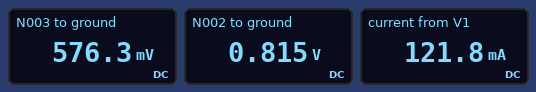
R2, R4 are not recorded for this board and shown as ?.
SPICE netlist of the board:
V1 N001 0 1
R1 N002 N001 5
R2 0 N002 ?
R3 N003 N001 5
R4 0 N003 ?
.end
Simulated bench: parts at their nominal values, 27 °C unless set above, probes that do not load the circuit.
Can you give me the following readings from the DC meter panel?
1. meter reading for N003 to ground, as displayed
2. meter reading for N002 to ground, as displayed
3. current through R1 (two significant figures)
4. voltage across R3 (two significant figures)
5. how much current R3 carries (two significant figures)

576.3 mV
0.815 V
37 mA
420 mV
85 mA
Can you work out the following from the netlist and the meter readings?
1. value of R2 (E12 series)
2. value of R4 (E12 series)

22 Ω
6.8 Ω
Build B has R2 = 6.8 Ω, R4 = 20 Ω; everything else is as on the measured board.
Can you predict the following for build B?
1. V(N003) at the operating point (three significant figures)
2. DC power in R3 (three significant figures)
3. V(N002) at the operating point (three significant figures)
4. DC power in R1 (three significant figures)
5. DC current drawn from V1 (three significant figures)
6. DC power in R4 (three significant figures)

800 mV
8.00 mW
576 mV
35.9 mW
125 mA
32.0 mW
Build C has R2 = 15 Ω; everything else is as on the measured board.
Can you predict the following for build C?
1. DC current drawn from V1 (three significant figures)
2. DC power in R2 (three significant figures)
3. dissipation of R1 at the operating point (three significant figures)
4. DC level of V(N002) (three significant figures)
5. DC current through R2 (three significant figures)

135 mA
37.5 mW
12.5 mW
750 mV
50.0 mA
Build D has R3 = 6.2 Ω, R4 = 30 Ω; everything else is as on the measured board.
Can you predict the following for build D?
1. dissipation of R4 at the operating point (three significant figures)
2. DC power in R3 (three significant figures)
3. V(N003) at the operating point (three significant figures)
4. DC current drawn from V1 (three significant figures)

22.9 mW
4.73 mW
829 mV
64.7 mA
